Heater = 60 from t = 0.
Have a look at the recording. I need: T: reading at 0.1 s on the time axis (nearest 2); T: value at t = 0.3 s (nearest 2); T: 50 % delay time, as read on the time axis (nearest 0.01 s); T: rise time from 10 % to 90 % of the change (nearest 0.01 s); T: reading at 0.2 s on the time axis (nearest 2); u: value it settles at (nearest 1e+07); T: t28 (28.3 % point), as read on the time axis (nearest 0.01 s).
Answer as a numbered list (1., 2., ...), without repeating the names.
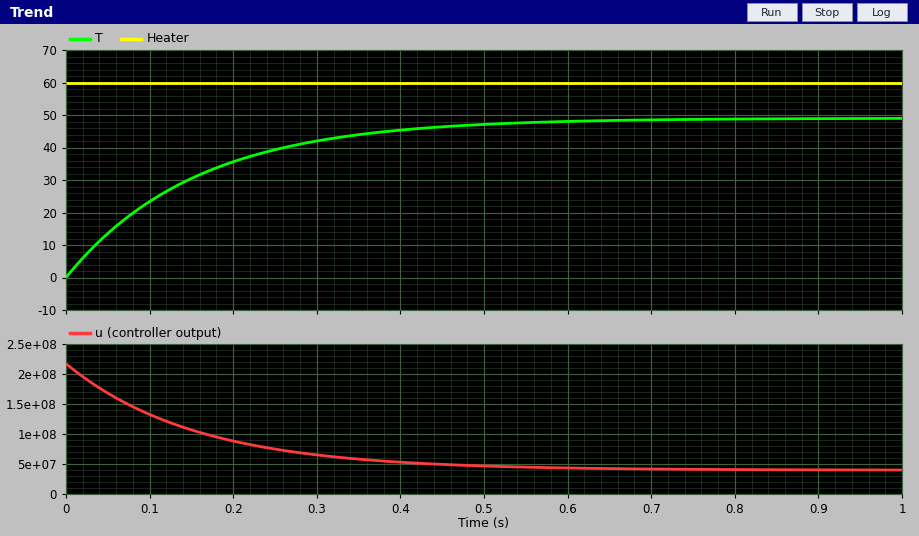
1. 24
2. 42
3. 0.11 s
4. 0.34 s
5. 36
6. 40000000
7. 0.05 s
